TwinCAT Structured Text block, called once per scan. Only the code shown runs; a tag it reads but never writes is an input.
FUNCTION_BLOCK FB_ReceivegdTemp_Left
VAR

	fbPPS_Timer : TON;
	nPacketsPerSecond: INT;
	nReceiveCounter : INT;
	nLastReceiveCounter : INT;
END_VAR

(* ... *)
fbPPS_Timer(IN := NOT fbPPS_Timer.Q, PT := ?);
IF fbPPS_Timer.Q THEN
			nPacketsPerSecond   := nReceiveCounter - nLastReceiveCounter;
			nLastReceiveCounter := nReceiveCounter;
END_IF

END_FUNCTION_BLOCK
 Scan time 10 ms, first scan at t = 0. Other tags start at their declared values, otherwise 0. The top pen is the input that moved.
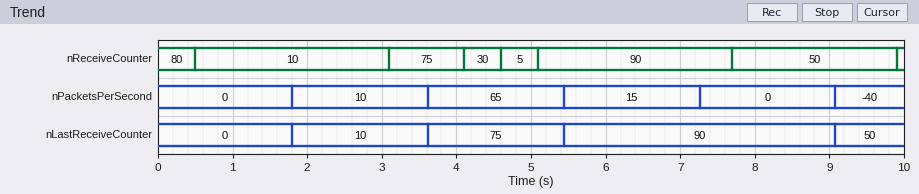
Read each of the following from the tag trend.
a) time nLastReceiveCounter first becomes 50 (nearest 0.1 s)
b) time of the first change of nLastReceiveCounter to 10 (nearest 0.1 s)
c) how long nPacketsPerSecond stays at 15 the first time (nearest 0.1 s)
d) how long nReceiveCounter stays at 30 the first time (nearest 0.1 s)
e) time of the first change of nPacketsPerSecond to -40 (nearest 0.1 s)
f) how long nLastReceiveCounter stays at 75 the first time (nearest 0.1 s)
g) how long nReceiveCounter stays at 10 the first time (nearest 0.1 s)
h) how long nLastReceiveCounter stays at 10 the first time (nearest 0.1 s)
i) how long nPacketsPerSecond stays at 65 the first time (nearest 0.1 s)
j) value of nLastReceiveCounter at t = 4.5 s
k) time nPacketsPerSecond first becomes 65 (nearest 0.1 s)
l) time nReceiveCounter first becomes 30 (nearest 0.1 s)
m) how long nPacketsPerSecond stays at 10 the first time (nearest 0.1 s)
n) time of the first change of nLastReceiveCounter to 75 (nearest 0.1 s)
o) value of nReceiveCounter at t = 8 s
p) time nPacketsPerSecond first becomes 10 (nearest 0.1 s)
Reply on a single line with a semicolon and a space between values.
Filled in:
9.1 s; 1.8 s; 1.8 s; 0.5 s; 9.1 s; 1.8 s; 2.6 s; 1.8 s; 1.8 s; 75; 3.6 s; 4.1 s; 1.8 s; 3.6 s; 50; 1.8 s
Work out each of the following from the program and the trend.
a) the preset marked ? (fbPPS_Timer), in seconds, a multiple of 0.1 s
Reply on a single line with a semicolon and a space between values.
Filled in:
1.8 s
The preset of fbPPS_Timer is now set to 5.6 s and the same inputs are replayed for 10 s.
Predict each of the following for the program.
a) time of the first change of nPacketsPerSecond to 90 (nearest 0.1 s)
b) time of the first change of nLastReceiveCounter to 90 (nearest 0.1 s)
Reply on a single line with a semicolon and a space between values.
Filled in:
5.6 s; 5.6 s
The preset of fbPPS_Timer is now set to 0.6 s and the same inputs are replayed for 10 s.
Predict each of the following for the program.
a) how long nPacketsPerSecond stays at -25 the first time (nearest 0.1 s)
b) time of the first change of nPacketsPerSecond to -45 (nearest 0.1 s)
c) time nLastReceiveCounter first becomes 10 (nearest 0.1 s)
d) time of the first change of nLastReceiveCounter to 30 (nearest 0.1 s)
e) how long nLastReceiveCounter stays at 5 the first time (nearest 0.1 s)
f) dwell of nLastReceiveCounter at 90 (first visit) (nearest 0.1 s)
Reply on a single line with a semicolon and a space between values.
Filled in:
0.6 s; 4.3 s; 0.6 s; 4.3 s; 0.6 s; 2.5 s
